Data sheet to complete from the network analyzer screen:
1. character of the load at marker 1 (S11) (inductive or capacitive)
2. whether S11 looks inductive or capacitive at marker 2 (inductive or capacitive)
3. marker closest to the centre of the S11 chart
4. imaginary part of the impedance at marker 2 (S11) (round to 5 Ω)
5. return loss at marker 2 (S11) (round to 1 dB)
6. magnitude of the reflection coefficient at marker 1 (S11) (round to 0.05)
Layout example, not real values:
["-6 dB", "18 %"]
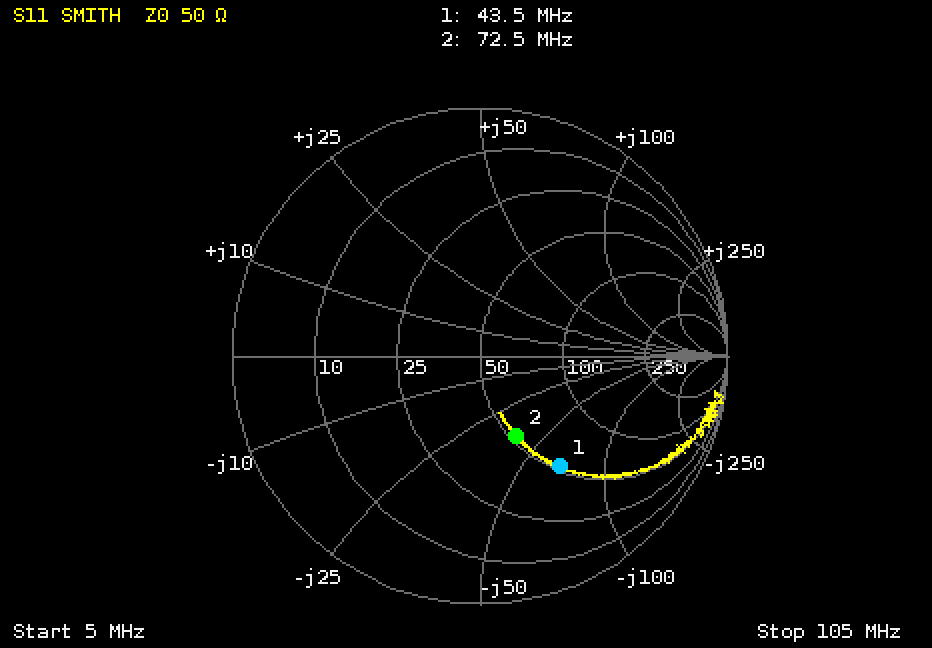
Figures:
["capacitive", "capacitive", "marker 2", "-40 Ω", "9 dB", "0.55"]
